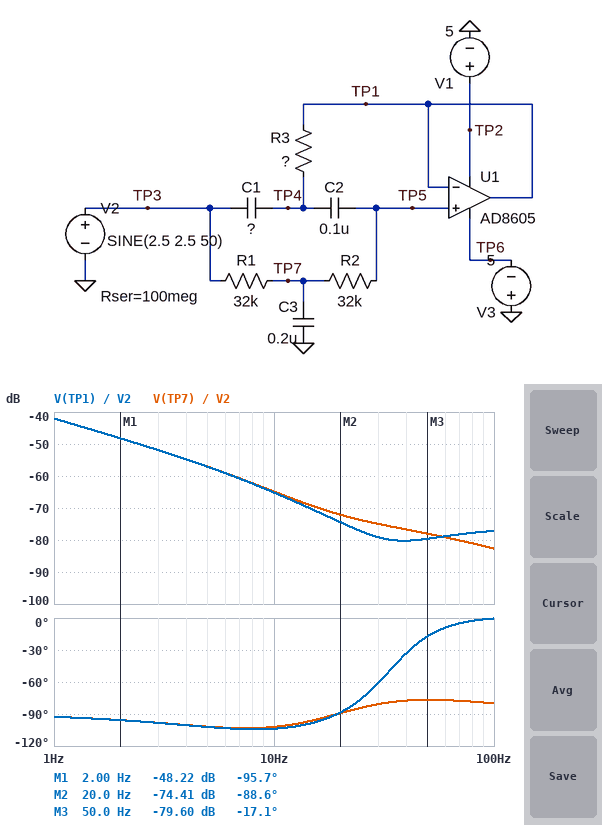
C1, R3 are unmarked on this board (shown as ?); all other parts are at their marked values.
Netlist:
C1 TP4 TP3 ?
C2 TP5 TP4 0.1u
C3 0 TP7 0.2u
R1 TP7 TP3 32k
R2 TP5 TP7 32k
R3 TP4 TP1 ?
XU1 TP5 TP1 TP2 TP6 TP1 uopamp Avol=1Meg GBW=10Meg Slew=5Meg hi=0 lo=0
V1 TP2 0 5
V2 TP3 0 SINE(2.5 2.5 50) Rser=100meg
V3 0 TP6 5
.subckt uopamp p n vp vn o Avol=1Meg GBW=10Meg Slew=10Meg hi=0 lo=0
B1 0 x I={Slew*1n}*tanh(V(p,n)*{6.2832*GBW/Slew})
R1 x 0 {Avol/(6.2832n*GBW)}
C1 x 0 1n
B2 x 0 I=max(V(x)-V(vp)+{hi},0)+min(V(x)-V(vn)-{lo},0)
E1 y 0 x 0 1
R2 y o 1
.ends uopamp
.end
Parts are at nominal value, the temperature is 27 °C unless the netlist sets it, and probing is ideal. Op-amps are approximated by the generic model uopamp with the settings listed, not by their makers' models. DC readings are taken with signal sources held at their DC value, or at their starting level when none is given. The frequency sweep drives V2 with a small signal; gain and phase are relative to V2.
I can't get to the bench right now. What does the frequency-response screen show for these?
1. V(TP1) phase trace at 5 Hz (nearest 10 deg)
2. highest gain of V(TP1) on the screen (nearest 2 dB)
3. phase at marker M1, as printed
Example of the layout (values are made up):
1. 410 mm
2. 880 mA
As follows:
1. -100 deg
2. -42 dB
3. -95.7 deg
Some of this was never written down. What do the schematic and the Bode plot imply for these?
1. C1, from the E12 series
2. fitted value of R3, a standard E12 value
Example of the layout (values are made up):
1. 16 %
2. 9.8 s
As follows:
1. 270 nF
2. 39 kΩ
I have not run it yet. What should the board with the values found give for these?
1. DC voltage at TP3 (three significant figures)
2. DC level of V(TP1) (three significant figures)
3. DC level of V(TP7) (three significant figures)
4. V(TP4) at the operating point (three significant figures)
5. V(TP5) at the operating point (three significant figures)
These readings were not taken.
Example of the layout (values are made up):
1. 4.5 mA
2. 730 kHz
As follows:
1. 2.50 V
2. 2.50 V
3. 2.50 V
4. 2.50 V
5. 2.50 V
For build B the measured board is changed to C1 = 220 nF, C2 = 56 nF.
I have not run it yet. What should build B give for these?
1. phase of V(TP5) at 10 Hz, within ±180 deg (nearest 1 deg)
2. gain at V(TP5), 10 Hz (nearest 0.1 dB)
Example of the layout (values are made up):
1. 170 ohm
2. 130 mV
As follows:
1. -105 deg
2. -64.3 dB
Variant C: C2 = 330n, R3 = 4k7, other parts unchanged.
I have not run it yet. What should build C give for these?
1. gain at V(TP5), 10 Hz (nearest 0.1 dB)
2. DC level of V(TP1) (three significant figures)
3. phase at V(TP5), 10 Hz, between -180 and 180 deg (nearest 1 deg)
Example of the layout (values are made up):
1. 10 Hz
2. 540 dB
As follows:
1. -64.0 dB
2. 2.50 V
3. -119 deg
